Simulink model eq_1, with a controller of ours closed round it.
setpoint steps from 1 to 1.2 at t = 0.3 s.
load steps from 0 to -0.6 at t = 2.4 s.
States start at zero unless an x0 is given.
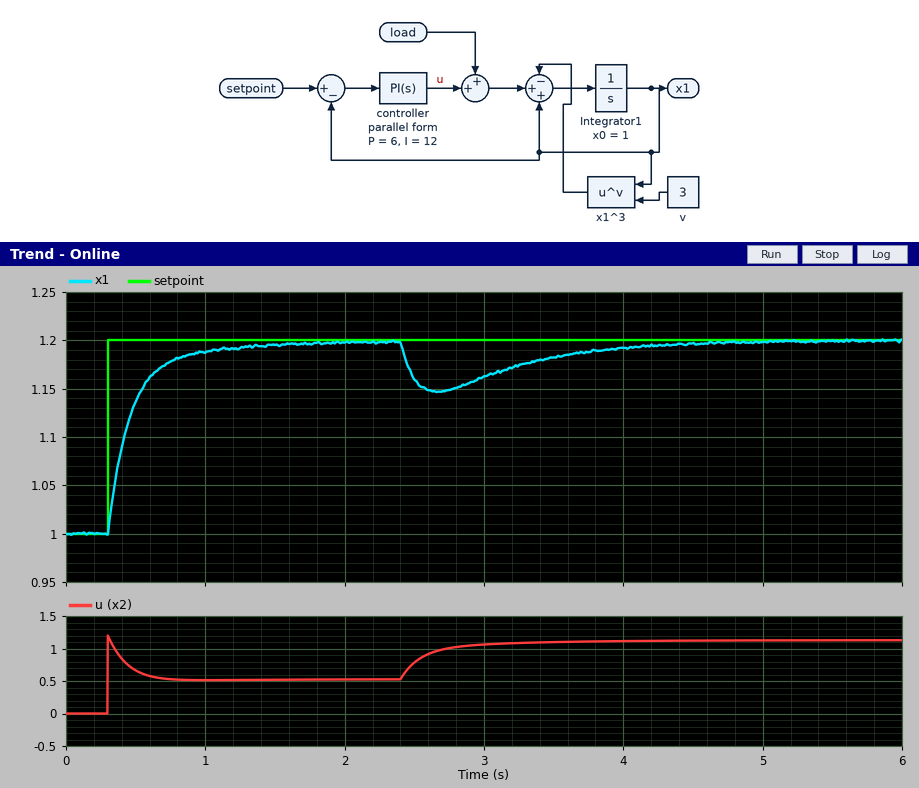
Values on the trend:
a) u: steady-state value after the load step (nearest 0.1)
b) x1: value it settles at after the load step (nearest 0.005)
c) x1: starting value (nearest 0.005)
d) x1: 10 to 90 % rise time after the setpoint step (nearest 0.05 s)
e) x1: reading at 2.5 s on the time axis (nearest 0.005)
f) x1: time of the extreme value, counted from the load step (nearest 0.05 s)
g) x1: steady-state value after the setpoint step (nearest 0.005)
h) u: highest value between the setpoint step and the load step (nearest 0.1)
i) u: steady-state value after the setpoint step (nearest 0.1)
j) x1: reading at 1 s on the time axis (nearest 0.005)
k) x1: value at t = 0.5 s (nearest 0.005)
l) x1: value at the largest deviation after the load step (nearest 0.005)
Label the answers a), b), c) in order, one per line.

a) 1.1
b) 1.200
c) 1.000
d) 0.45 s
e) 1.160
f) 0.25 s
g) 1.200
h) 1.2
i) 0.5
j) 1.190
k) 1.135
l) 1.145
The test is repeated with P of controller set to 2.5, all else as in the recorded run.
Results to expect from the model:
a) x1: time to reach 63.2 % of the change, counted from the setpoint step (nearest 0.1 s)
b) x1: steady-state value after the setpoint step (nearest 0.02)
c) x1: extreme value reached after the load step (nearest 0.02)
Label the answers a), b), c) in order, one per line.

a) 0.3 s
b) 1.20
c) 1.12
